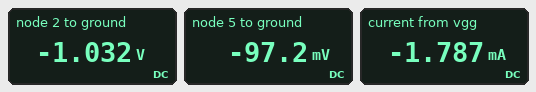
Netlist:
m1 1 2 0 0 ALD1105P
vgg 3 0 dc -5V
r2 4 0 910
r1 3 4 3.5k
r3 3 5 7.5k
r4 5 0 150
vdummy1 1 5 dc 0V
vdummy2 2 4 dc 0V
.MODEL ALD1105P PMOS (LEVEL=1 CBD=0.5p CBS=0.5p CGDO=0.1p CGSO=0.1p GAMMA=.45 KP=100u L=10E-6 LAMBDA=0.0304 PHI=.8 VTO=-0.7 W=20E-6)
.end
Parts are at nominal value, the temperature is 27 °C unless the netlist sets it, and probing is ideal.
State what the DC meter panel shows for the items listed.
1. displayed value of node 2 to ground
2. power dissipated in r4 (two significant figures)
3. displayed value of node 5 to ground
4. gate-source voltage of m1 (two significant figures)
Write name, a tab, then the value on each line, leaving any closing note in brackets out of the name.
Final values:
displayed value of node 2 to ground	-1.032 V
power dissipated in r4	63 µW
displayed value of node 5 to ground	-97.2 mV
gate-source voltage of m1	-1.0 V
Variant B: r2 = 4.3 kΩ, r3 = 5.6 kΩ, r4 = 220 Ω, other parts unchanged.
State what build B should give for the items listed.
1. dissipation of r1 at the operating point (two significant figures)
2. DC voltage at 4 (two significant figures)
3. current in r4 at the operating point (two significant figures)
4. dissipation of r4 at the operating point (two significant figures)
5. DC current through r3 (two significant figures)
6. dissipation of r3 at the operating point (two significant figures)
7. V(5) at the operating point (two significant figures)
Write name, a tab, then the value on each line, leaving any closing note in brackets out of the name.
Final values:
dissipation of r1 at the operating point	1.4 mW
DC voltage at 4	-2.8 V
current in r4 at the operating point	790 µA
dissipation of r4 at the operating point	140 µW
DC current through r3	860 µA
dissipation of r3 at the operating point	4.2 mW
V(5) at the operating point	-170 mV
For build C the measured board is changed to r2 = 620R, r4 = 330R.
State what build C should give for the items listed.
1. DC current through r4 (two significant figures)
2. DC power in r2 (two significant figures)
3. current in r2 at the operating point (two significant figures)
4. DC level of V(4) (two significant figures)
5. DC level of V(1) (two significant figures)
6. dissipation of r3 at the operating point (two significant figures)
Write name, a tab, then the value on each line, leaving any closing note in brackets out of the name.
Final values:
DC current through r4	640 µA
DC power in r2	910 µW
current in r2 at the operating point	1.2 mA
DC level of V(4)	-750 mV
DC level of V(1)	-210 mV
dissipation of r3 at the operating point	3.1 mW
